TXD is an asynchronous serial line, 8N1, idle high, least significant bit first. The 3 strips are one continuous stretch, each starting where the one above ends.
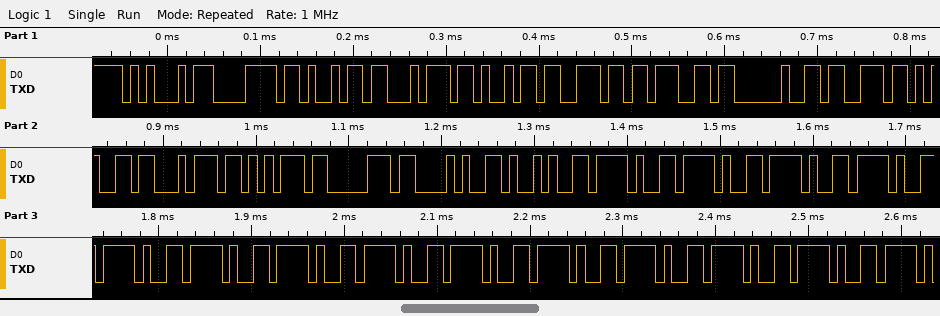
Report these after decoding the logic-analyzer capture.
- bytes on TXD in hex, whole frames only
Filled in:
45 78 69 74 69 6E 67 20 73 65 74 75 70 28 29 2F 2F 2F 2F 2F 2F 2F 2F 2F 2F 2F 2F 2F
